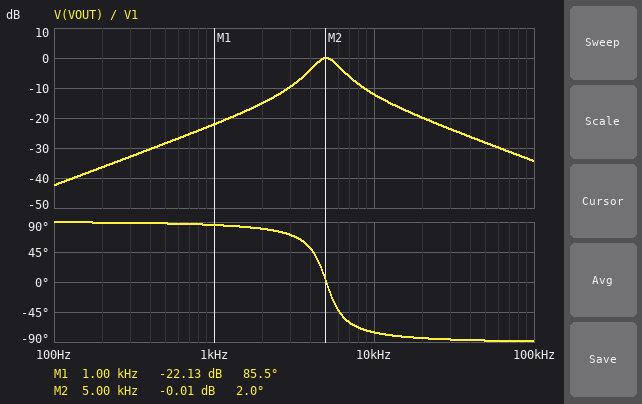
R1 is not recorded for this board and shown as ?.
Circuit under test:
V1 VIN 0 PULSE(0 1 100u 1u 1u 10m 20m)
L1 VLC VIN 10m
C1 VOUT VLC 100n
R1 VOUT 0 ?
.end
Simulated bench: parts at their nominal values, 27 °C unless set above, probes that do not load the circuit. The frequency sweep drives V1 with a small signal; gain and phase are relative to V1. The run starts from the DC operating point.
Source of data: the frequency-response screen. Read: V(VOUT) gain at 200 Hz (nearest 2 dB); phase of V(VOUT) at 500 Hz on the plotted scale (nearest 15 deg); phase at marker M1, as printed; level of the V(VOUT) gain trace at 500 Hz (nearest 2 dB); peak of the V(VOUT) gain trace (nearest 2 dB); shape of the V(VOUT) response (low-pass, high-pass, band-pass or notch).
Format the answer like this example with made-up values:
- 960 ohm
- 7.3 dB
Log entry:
- -36 dB
- 90 deg
- 85.5 deg
- -28 dB
- 0 dB
- band-pass
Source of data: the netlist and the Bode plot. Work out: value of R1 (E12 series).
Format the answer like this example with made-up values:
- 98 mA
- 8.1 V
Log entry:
- 120 Ω
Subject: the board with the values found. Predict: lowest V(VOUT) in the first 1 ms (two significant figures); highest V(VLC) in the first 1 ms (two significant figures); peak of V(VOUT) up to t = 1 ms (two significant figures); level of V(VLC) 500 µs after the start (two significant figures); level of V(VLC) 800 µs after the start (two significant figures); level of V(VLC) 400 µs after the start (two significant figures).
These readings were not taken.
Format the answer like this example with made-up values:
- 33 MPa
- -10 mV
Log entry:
- -160 mV
- 1.6 V
- 290 mV
- 910 mV
- 1.0 V
- 1.2 V
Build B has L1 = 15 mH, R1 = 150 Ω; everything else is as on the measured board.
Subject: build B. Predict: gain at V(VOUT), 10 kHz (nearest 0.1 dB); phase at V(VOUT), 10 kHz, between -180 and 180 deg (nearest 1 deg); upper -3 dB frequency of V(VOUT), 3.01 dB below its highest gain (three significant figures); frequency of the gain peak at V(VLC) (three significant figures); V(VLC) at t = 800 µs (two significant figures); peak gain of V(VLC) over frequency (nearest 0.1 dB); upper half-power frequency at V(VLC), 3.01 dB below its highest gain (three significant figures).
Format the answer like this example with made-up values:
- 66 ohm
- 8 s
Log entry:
- -14.5 dB
- -79 deg
- 4.98 kHz
- 3.97 kHz
- 980 mV
- 9.0 dB
- 4.73 kHz
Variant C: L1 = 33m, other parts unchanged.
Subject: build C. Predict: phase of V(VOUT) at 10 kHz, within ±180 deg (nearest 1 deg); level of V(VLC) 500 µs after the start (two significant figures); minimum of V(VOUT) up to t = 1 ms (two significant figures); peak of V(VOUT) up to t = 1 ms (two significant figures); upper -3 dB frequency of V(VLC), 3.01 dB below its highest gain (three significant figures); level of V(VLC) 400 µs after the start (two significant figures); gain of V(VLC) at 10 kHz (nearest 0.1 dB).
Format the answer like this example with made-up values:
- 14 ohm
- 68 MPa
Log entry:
- -86 deg
- 640 mV
- -130 mV
- 180 mV
- 3.02 kHz
- 680 mV
- -19.7 dB
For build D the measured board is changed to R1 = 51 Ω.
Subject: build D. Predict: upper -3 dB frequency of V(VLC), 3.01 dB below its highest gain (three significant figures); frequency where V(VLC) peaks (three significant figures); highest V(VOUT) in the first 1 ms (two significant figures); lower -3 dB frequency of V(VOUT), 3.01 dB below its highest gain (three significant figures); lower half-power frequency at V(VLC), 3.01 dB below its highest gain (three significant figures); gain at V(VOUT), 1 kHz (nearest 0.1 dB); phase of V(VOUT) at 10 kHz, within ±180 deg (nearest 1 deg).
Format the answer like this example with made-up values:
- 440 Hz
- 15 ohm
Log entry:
- 5.39 kHz
- 5.00 kHz
- 140 mV
- 4.64 kHz
- 4.58 kHz
- -29.5 dB
- -84 deg
